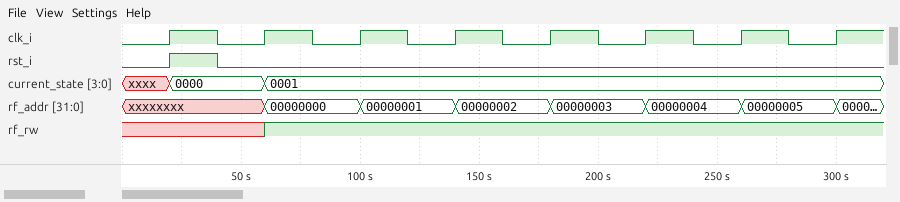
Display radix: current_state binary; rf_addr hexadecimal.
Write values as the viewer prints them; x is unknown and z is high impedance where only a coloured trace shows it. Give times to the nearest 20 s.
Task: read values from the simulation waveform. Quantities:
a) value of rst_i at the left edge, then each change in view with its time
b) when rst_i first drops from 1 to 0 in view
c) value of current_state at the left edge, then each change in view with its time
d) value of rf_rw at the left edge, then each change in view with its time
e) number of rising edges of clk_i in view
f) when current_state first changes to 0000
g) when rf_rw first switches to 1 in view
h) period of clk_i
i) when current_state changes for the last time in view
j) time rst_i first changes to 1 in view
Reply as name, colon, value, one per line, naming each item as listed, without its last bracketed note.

value of rst_i at the left edge, then each change in view with its time: 0, 1 at 20 s, 0 at 40 s
when rst_i first drops from 1 to 0 in view: 40 s
value of current_state at the left edge, then each change in view with its time: xxxx, 0000 at 20 s, 0001 at 60 s
value of rf_rw at the left edge, then each change in view with its time: x, 1 at 60 s
number of rising edges of clk_i in view: 8
when current_state first changes to 0000: 20 s
when rf_rw first switches to 1 in view: 60 s
period of clk_i: 40 s
when current_state changes for the last time in view: 60 s
time rst_i first changes to 1 in view: 20 s
